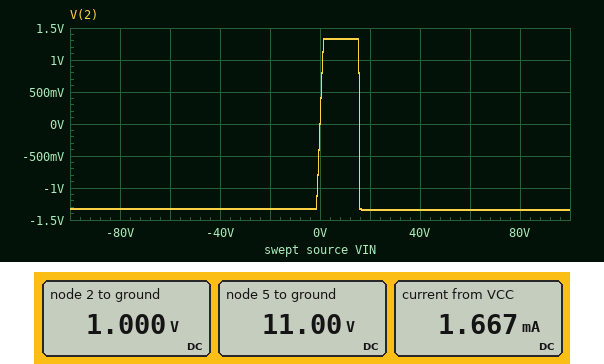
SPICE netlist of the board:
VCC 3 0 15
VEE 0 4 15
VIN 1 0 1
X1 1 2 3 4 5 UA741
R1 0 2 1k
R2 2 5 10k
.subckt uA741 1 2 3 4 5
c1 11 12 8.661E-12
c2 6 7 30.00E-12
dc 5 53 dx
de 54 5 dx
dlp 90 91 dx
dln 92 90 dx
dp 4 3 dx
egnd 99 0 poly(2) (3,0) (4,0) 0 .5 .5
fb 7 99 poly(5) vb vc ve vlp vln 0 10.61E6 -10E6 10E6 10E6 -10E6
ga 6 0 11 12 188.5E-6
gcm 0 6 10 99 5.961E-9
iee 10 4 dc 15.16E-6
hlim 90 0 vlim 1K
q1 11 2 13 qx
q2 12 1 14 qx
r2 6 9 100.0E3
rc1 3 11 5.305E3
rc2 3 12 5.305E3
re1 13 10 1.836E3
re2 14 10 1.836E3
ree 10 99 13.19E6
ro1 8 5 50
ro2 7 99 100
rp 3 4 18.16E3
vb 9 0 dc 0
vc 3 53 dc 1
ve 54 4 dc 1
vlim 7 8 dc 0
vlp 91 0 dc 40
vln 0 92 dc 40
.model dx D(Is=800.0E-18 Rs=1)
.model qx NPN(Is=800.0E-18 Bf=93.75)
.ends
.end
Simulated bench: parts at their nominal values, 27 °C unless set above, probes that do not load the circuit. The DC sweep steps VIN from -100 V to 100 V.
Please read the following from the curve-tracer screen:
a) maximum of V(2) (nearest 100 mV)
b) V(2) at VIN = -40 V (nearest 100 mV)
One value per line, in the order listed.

1.3 V
-1.3 V
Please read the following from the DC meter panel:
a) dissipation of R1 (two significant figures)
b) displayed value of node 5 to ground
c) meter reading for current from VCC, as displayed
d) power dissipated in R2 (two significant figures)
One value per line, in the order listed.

1.0 mW
11.00 V
1.667 mA
10 mW
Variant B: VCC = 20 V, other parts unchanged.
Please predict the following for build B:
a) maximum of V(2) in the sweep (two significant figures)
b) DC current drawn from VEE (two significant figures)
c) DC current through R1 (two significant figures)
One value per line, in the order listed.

1.8 V
1.9 mA
1.0 mA
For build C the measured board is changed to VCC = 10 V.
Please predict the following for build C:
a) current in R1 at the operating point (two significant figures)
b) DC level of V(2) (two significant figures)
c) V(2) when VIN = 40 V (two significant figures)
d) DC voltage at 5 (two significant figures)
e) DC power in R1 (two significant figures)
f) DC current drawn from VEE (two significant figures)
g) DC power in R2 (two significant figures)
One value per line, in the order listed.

870 µA
870 mV
-1.3 V
9.6 V
760 µW
1.4 mA
7.6 mW
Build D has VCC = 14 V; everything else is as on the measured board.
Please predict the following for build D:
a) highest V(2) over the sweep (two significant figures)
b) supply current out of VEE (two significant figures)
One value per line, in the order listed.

1.2 V
1.6 mA
